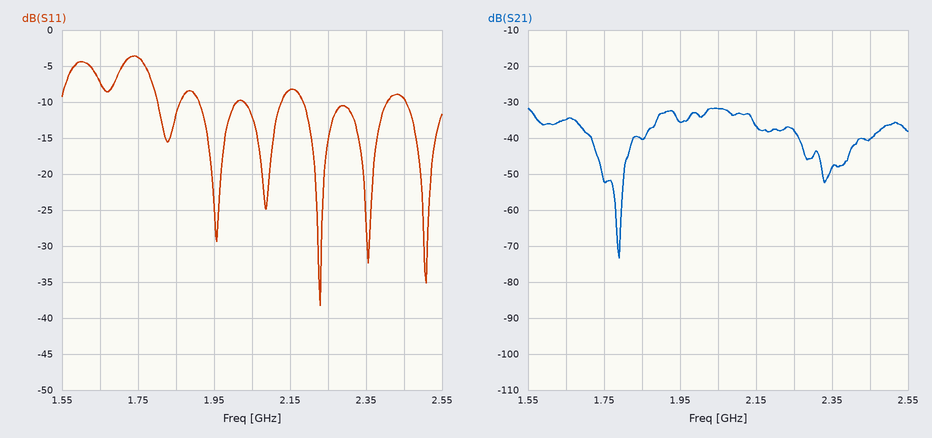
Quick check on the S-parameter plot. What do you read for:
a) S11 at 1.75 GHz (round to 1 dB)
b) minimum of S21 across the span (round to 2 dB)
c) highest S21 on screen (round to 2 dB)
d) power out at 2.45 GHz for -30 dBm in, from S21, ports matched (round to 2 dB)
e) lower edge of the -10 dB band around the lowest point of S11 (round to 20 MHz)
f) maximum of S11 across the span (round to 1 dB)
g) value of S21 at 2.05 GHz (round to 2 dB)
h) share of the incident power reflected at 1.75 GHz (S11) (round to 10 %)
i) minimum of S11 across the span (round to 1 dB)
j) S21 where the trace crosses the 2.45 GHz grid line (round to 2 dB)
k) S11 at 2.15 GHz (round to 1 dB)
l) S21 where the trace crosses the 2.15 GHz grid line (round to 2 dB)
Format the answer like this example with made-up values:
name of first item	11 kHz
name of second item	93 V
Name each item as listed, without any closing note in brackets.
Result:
S11 at 1.75 GHz	-4 dB
minimum of S21 across the span	-74 dB
highest S21 on screen	-32 dB
power out at 2.45 GHz for -30 dBm in, from S21, ports matched	-70 dBm
lower edge of the -10 dB band around the lowest point of S11	2.18 GHz
maximum of S11 across the span	-4 dB
value of S21 at 2.05 GHz	-32 dB
share of the incident power reflected at 1.75 GHz (S11)	40 %
minimum of S11 across the span	-38 dB
S21 where the trace crosses the 2.45 GHz grid line	-40 dB
S11 at 2.15 GHz	-8 dB
S21 where the trace crosses the 2.15 GHz grid line	-36 dB
